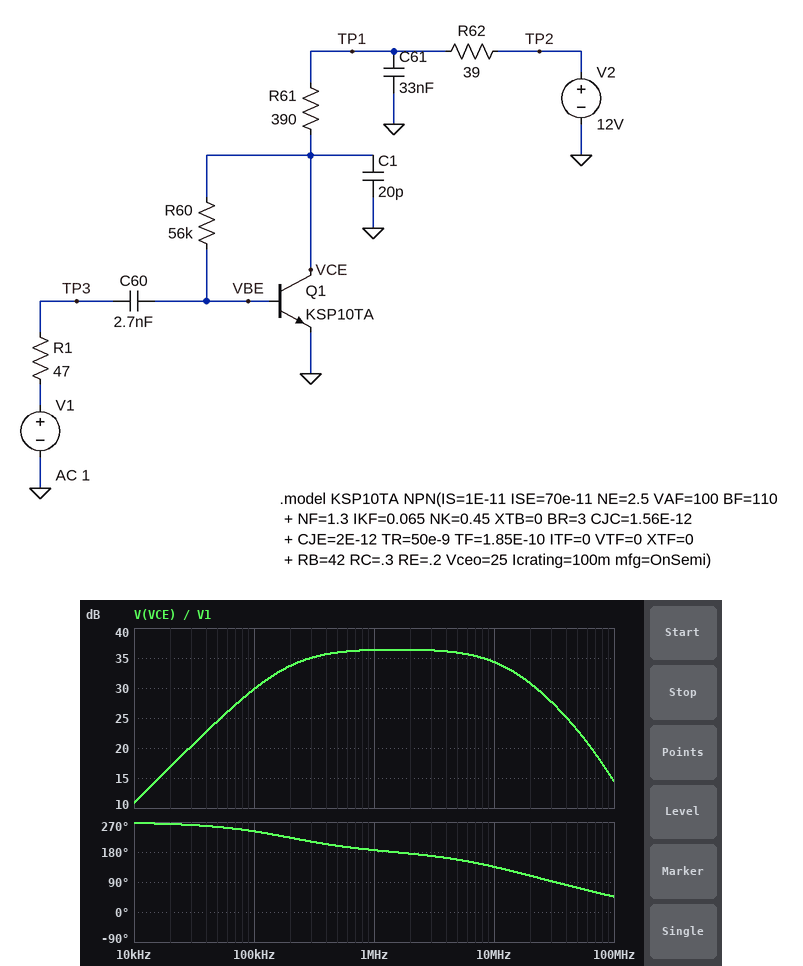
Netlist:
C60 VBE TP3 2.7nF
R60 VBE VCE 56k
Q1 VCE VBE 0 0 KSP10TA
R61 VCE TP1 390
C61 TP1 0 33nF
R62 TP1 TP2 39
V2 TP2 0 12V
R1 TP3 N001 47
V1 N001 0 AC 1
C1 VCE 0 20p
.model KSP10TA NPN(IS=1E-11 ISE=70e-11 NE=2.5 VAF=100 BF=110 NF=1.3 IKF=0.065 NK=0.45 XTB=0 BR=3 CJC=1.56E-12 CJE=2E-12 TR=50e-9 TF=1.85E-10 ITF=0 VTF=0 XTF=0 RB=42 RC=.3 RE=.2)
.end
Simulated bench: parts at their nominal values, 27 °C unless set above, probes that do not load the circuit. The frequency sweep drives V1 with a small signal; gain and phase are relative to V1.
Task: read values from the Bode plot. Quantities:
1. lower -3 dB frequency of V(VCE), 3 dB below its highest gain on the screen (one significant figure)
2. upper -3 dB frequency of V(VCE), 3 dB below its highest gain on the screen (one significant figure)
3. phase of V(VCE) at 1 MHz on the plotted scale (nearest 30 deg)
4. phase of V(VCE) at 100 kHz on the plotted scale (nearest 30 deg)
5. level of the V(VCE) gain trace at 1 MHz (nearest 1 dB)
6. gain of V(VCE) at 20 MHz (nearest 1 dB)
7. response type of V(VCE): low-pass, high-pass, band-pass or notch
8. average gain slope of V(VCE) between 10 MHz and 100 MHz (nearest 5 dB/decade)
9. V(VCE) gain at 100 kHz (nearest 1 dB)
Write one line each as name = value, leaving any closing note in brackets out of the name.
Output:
lower -3 dB frequency of V(VCE), 3 dB below its highest gain on the screen = 200 kHz
upper -3 dB frequency of V(VCE), 3 dB below its highest gain on the screen = 10 MHz
phase of V(VCE) at 1 MHz on the plotted scale = 180 deg
phase of V(VCE) at 100 kHz on the plotted scale = 240 deg
level of the V(VCE) gain trace at 1 MHz = 36 dB
gain of V(VCE) at 20 MHz = 31 dB
response type of V(VCE): low-pass, high-pass, band-pass or notch = band-pass
average gain slope of V(VCE) between 10 MHz and 100 MHz = -20 dB/decade
V(VCE) gain at 100 kHz = 30 dB
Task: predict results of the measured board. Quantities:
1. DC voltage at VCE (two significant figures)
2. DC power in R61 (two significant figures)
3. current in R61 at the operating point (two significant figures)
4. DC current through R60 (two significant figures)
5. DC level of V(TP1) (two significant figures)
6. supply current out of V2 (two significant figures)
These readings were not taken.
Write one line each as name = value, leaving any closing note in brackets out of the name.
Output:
DC voltage at VCE = 7.8 V
DC power in R61 = 38 mW
current in R61 at the operating point = 9.8 mA
DC current through R60 = 130 µA
DC level of V(TP1) = 12 V
supply current out of V2 = 9.8 mA
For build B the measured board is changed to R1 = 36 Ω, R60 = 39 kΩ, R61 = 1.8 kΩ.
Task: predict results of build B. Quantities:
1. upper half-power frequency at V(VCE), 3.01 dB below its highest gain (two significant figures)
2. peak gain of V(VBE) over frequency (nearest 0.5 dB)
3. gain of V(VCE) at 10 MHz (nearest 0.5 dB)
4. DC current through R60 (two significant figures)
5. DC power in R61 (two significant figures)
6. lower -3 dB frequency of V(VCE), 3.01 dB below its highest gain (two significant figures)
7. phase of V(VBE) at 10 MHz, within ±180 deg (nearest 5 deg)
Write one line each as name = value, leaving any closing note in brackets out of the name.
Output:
upper half-power frequency at V(VCE), 3.01 dB below its highest gain = 4.5 MHz
peak gain of V(VBE) over frequency = -1.5 dB
gain of V(VCE) at 10 MHz = 35.0 dB
DC current through R60 = 67 µA
DC power in R61 = 40 mW
lower -3 dB frequency of V(VCE), 3.01 dB below its highest gain = 270 kHz
phase of V(VBE) at 10 MHz, within ±180 deg = 0 deg
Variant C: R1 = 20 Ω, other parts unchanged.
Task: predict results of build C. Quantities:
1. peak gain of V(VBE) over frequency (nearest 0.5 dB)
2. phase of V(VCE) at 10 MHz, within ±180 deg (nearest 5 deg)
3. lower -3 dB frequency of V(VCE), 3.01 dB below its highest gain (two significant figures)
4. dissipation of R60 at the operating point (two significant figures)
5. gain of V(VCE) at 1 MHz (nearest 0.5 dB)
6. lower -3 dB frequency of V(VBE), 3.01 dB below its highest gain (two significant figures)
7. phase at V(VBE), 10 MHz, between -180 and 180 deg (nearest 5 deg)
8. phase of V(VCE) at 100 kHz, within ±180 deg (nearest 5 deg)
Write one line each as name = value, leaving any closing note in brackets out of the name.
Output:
peak gain of V(VBE) over frequency = -1.0 dB
phase of V(VCE) at 10 MHz, within ±180 deg = 140 deg
lower -3 dB frequency of V(VCE), 3.01 dB below its highest gain = 210 kHz
dissipation of R60 at the operating point = 890 µW
gain of V(VCE) at 1 MHz = 37.0 dB
lower -3 dB frequency of V(VBE), 3.01 dB below its highest gain = 220 kHz
phase at V(VBE), 10 MHz, between -180 and 180 deg = 0 deg
phase of V(VCE) at 100 kHz, within ±180 deg = -115 deg
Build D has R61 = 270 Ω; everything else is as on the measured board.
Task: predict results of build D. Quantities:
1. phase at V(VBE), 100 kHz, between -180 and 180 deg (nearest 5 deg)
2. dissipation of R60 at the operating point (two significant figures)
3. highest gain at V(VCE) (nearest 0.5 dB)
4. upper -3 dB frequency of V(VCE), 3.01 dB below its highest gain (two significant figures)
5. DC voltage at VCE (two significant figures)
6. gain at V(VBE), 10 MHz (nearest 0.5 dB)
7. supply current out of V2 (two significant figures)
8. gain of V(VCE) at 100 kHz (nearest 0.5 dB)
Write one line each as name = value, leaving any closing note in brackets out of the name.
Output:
phase at V(VBE), 100 kHz, between -180 and 180 deg = 65 deg
dissipation of R60 at the operating point = 1.1 mW
highest gain at V(VCE) = 34.0 dB
upper -3 dB frequency of V(VCE), 3.01 dB below its highest gain = 16 MHz
DC voltage at VCE = 8.6 V
gain at V(VBE), 10 MHz = -2.0 dB
supply current out of V2 = 11 mA
gain of V(VCE) at 100 kHz = 28.0 dB
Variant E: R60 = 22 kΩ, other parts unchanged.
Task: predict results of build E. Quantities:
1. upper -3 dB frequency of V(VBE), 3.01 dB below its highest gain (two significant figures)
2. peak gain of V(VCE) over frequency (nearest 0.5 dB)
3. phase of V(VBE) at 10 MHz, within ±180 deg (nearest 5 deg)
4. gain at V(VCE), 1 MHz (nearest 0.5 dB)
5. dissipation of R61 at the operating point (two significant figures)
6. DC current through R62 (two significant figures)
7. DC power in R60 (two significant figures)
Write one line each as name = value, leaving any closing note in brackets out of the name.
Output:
upper -3 dB frequency of V(VBE), 3.01 dB below its highest gain = 330 MHz
peak gain of V(VCE) over frequency = 37.5 dB
phase of V(VBE) at 10 MHz, within ±180 deg = 0 deg
gain at V(VCE), 1 MHz = 37.0 dB
dissipation of R61 at the operating point = 96 mW
DC current through R62 = 16 mA
DC power in R60 = 940 µW
